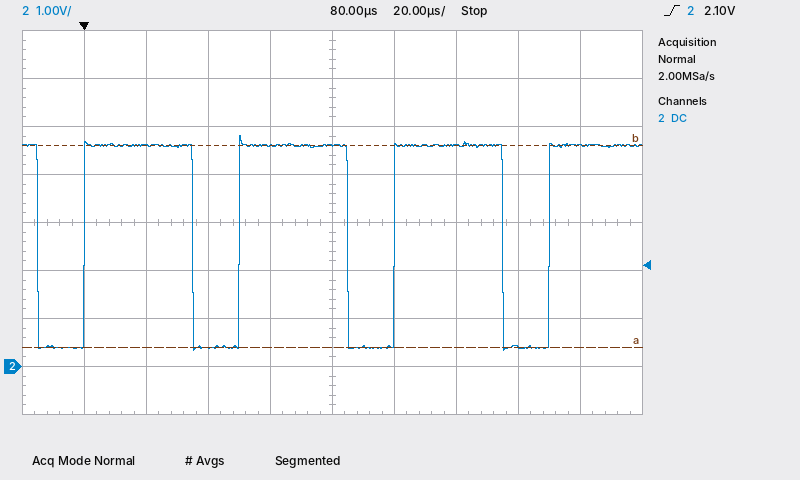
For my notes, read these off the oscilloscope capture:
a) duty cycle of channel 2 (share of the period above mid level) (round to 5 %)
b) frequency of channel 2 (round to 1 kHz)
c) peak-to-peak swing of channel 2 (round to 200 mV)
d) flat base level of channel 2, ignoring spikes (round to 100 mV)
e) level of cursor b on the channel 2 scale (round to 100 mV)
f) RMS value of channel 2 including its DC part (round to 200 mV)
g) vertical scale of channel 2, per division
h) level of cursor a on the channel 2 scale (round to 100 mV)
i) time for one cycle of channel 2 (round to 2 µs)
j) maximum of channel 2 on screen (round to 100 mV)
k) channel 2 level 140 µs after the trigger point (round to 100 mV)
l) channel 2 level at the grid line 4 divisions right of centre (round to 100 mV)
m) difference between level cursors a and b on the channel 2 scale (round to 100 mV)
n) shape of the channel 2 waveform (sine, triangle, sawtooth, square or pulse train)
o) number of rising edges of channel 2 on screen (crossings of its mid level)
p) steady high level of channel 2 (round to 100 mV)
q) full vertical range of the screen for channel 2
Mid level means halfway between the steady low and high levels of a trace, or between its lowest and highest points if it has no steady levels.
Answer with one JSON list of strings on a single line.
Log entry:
["70 %", "20 kHz", "4.4 V", "400 mV", "4.6 V", "3.8 V", "1 V", "400 mV", "50 µs", "4.8 V", "400 mV", "4.6 V", "4.2 V", "pulse train", "4", "4.6 V", "8 V"]
